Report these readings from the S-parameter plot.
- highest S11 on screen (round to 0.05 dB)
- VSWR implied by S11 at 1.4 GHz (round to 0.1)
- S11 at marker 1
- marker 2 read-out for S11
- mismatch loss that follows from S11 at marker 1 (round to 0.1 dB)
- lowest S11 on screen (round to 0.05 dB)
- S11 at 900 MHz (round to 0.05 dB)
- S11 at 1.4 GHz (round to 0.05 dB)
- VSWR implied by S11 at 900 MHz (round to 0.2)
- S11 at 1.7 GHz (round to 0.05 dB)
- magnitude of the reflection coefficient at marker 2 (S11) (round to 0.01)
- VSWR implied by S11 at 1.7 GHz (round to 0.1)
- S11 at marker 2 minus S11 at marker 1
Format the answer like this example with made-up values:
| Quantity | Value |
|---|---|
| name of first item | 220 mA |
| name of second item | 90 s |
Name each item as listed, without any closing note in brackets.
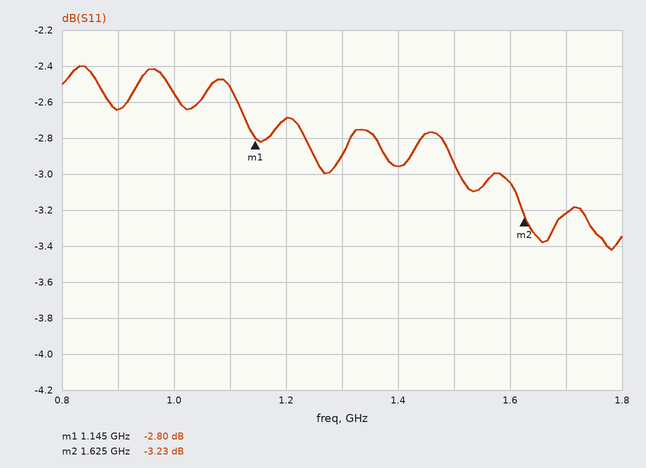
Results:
| Quantity | Value |
|---|---|
| highest S11 on screen | -2.40 dB |
| VSWR implied by S11 at 1.4 GHz | 5.9 |
| S11 at marker 1 | -2.80 dB |
| marker 2 read-out for S11 | -3.23 dB |
| mismatch loss that follows from S11 at marker 1 | 3.2 dB |
| lowest S11 on screen | -3.40 dB |
| S11 at 900 MHz | -2.65 dB |
| S11 at 1.4 GHz | -2.95 dB |
| VSWR implied by S11 at 900 MHz | 6.6 |
| S11 at 1.7 GHz | -3.20 dB |
| magnitude of the reflection coefficient at marker 2 (S11) | 0.69 |
| VSWR implied by S11 at 1.7 GHz | 5.5 |
| S11 at marker 2 minus S11 at marker 1 | -0.43 dB |
